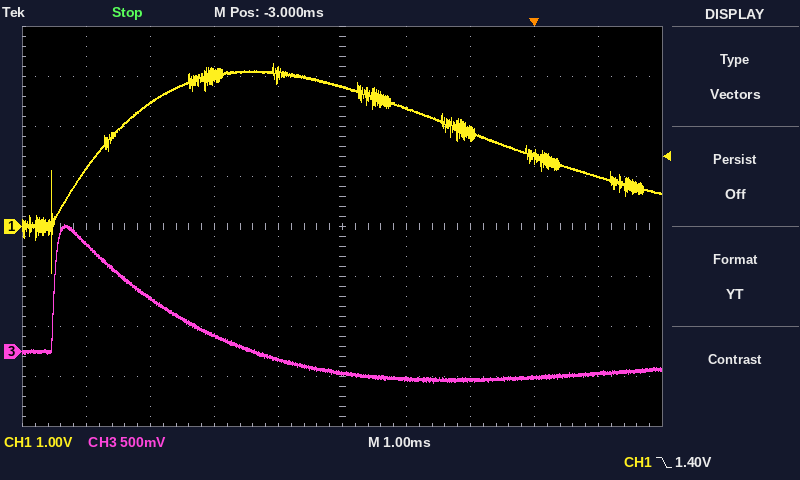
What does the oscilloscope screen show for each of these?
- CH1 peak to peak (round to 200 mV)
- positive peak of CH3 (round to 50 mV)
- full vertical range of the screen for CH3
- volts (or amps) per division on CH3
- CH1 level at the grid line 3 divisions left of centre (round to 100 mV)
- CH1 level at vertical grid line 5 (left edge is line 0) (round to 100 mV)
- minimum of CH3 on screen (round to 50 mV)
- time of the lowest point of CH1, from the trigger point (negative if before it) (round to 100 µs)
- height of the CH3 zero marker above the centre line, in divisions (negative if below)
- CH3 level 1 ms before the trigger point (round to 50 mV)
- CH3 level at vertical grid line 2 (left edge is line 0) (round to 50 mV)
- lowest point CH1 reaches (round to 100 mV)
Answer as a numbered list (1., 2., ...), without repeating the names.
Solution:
1. 4.2 V
2. 1.25 V
3. 4 V
4. 500 mV
5. 2.5 V
6. 2.8 V
7. -300 mV
8. -7.5 ms
9. -2.5 div
10. -300 mV
11. 550 mV
12. -900 mV
